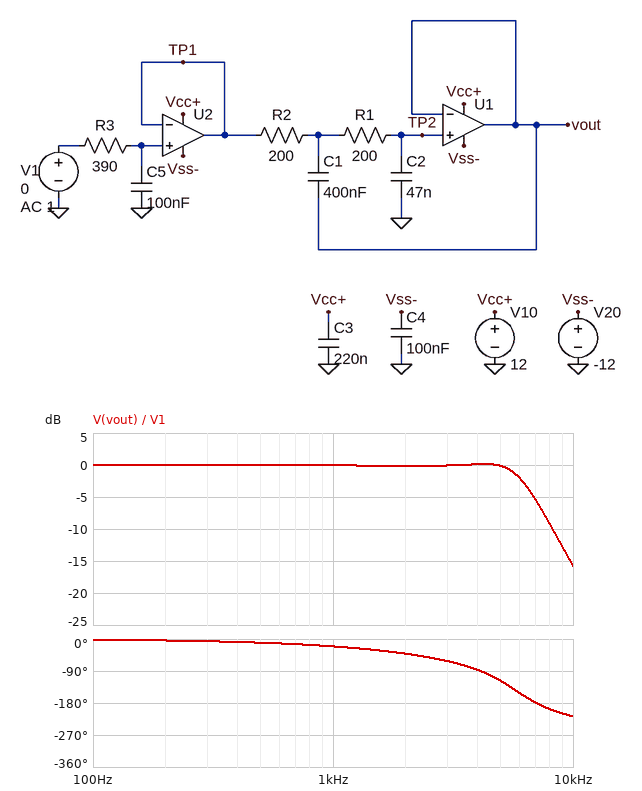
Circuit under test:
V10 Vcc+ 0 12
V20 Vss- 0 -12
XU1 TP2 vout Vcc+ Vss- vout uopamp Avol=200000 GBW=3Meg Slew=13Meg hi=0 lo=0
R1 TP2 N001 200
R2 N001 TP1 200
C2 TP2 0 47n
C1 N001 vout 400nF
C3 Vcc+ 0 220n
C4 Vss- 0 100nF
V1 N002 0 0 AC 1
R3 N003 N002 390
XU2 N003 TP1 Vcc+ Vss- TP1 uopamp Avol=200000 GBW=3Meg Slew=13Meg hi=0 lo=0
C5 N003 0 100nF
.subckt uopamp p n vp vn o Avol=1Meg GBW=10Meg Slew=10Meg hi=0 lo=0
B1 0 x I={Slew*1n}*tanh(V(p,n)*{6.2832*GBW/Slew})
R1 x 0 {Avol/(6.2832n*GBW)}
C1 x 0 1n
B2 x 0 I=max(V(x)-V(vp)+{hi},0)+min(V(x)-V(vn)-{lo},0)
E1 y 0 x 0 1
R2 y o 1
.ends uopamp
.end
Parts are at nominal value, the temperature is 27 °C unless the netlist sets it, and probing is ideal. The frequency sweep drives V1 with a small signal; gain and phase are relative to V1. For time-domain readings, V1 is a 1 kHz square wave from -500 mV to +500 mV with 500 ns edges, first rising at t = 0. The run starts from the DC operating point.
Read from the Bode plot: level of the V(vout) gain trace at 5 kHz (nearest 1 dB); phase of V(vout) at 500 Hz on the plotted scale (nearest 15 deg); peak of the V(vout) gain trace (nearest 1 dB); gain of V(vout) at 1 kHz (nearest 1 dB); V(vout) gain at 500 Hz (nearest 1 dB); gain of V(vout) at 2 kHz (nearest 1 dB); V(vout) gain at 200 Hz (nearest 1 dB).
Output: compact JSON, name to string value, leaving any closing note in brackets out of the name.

{"level of the V(vout) gain trace at 5 kHz": "0 dB", "phase of V(vout) at 500 Hz on the plotted scale": "-15 deg", "peak of the V(vout) gain trace": "0 dB", "gain of V(vout) at 1 kHz": "0 dB", "V(vout) gain at 500 Hz": "0 dB", "gain of V(vout) at 2 kHz": "0 dB", "V(vout) gain at 200 Hz": "0 dB"}
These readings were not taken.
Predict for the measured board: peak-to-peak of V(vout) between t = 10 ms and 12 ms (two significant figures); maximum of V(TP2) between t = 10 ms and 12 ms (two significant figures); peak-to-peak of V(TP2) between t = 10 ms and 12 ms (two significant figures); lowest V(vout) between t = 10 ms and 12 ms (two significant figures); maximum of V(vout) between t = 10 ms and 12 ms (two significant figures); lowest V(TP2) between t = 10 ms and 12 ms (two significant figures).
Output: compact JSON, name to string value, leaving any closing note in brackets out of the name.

{"peak-to-peak of V(vout) between t = 10 ms and 12 ms": "1.2 V", "maximum of V(TP2) between t = 10 ms and 12 ms": "610 mV", "peak-to-peak of V(TP2) between t = 10 ms and 12 ms": "1.2 V", "lowest V(vout) between t = 10 ms and 12 ms": "-610 mV", "maximum of V(vout) between t = 10 ms and 12 ms": "610 mV", "lowest V(TP2) between t = 10 ms and 12 ms": "-610 mV"}
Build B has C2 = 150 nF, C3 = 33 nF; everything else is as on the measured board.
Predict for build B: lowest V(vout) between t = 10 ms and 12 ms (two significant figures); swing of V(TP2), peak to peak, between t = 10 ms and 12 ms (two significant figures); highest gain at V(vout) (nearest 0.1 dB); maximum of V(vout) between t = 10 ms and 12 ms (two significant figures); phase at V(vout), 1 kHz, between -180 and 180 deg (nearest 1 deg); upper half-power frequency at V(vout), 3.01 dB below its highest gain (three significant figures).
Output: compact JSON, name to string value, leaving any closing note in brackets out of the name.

{"lowest V(vout) between t = 10 ms and 12 ms": "-550 mV", "swing of V(TP2), peak to peak, between t = 10 ms and 12 ms": "1.1 V", "highest gain at V(vout)": "0 dB", "maximum of V(vout) between t = 10 ms and 12 ms": "550 mV", "phase at V(vout), 1 kHz, between -180 and 180 deg": "-36 deg", "upper half-power frequency at V(vout), 3.01 dB below its highest gain": "3.00 kHz"}
